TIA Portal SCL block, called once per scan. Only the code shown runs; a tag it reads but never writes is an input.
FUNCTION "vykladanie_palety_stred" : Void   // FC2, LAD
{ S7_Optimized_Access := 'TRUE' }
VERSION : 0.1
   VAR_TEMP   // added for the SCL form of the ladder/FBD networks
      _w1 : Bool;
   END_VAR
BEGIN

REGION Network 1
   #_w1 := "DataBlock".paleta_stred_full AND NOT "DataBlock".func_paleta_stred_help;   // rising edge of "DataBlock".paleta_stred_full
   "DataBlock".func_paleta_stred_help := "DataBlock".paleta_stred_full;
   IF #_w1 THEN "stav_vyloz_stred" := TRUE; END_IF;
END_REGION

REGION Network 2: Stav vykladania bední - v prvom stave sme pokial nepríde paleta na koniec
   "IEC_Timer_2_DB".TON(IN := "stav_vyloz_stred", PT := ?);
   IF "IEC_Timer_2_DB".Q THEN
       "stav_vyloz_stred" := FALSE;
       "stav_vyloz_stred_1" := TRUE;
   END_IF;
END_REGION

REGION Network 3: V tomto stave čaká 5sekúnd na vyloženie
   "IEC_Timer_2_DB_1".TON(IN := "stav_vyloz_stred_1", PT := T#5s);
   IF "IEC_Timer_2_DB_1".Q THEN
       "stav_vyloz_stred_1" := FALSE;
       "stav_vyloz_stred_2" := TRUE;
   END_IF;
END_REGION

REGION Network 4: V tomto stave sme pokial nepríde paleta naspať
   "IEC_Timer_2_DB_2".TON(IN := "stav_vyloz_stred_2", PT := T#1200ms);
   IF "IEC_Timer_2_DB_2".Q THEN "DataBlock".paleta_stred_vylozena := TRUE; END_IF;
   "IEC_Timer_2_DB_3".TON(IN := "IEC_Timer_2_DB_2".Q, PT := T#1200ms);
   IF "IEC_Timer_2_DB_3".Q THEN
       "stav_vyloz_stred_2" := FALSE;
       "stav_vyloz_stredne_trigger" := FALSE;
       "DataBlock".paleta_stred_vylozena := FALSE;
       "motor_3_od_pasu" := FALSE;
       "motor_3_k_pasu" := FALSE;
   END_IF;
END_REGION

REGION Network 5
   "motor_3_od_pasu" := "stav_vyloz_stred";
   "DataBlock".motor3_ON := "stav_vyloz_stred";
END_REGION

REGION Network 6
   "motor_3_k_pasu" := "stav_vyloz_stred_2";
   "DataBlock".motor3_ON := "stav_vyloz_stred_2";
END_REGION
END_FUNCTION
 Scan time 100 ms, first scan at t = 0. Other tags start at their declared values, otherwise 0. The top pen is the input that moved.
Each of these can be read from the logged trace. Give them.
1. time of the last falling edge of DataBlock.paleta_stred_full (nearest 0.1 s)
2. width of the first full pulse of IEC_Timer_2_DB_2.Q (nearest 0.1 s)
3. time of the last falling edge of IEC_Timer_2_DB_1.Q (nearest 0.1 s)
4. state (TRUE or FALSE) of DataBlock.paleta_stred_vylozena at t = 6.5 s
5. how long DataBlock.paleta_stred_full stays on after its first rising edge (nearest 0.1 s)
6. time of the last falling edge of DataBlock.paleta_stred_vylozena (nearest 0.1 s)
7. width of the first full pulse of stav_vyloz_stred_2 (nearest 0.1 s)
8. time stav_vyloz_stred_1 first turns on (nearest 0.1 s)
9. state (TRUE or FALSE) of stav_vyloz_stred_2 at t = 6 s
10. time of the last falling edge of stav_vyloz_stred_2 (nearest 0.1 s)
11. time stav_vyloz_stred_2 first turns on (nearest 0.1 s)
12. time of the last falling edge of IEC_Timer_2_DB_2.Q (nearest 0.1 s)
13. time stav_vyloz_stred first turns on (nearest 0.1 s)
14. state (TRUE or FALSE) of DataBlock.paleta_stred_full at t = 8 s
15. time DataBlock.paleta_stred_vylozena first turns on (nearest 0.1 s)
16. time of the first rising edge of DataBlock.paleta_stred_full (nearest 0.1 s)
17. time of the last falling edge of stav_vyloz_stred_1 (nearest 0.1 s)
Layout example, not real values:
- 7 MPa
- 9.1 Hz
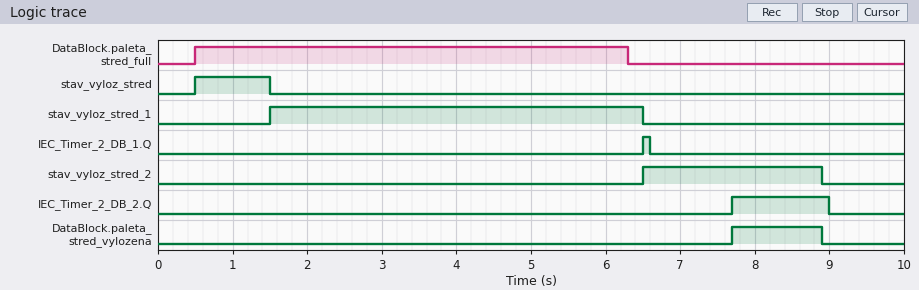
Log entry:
- 6.3 s
- 1.3 s
- 6.6 s
- FALSE
- 5.8 s
- 8.9 s
- 2.4 s
- 1.5 s
- FALSE
- 8.9 s
- 6.5 s
- 9.0 s
- 0.5 s
- FALSE
- 7.7 s
- 0.5 s
- 6.5 s
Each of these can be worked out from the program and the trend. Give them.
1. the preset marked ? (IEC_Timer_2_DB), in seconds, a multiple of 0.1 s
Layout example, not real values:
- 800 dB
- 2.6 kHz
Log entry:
- 1.0 s
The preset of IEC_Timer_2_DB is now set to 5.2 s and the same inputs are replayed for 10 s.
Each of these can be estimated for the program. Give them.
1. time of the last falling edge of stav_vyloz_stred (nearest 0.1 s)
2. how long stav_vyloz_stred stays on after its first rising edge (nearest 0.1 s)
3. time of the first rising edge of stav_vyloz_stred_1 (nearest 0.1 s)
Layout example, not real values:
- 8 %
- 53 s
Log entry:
- 5.7 s
- 5.2 s
- 5.7 s
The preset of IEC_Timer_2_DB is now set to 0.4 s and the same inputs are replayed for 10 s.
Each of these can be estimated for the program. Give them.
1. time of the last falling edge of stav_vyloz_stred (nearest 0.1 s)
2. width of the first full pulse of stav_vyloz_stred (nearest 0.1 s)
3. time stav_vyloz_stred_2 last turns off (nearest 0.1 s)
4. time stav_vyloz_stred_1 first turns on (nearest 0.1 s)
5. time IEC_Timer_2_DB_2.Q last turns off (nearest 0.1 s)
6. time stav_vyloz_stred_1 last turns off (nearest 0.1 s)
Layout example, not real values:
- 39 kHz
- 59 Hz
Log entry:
- 0.9 s
- 0.4 s
- 8.3 s
- 0.9 s
- 8.4 s
- 5.9 s
